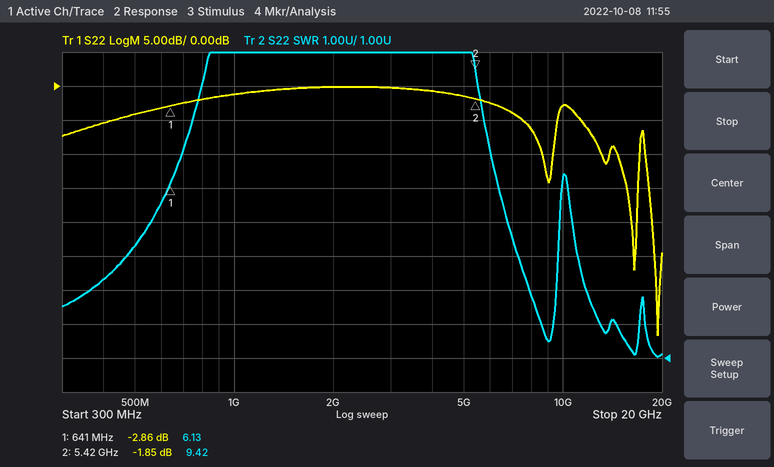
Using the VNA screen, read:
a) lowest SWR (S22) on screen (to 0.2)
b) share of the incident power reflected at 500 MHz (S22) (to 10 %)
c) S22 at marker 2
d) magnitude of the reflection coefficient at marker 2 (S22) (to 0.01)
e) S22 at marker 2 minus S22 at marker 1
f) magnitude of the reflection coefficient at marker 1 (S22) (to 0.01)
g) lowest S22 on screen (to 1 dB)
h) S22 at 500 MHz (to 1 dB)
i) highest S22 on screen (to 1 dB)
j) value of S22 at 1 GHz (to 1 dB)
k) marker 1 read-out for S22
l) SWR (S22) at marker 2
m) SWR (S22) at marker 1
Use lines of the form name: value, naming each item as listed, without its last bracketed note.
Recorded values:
lowest SWR (S22) on screen: 1.0
share of the incident power reflected at 500 MHz (S22): 40 %
S22 at marker 2: -1.85 dB
magnitude of the reflection coefficient at marker 2 (S22): 0.81
S22 at marker 2 minus S22 at marker 1: 1.01 dB
magnitude of the reflection coefficient at marker 1 (S22): 0.72
lowest S22 on screen: -37 dB
S22 at 500 MHz: -4 dB
highest S22 on screen: 0 dB
value of S22 at 1 GHz: -1 dB
marker 1 read-out for S22: -2.86 dB
SWR (S22) at marker 2: 9.42
SWR (S22) at marker 1: 6.13
